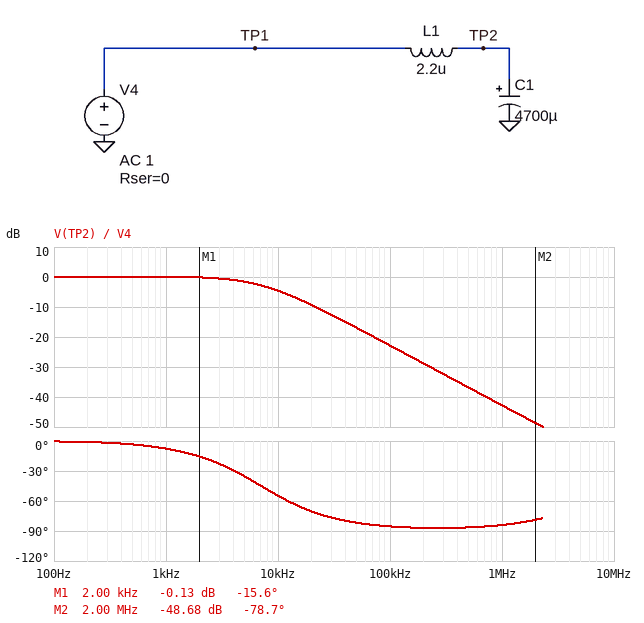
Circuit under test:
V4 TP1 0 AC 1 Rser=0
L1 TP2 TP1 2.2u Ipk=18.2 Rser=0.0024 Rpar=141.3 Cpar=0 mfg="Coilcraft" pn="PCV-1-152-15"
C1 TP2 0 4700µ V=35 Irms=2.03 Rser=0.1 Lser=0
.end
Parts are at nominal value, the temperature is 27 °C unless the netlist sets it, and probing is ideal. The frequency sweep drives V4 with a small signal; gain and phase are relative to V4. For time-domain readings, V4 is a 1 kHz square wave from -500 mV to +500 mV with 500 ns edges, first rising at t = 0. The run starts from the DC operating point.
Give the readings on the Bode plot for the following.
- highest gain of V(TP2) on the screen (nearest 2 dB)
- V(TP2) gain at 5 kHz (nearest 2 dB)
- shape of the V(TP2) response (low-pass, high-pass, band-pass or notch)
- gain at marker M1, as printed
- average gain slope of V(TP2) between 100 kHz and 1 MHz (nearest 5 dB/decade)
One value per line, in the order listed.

0 dB
-2 dB
low-pass
-0.13 dB
-20 dB/decade
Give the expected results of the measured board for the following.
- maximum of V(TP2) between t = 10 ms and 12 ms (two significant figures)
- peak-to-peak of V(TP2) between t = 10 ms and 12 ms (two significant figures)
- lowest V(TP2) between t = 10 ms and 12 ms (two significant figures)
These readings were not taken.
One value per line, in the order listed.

510 mV
1.0 V
-510 mV
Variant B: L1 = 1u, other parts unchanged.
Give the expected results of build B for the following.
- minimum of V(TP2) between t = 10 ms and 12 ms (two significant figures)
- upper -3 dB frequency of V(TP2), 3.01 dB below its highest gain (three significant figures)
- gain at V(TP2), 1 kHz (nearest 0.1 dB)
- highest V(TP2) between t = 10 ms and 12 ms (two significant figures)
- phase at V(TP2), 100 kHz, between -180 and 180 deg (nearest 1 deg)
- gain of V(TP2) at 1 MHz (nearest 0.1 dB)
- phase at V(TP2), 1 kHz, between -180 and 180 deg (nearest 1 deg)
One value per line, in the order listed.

-500 mV
15.9 kHz
0 dB
500 mV
-81 deg
-36.0 dB
-4 deg
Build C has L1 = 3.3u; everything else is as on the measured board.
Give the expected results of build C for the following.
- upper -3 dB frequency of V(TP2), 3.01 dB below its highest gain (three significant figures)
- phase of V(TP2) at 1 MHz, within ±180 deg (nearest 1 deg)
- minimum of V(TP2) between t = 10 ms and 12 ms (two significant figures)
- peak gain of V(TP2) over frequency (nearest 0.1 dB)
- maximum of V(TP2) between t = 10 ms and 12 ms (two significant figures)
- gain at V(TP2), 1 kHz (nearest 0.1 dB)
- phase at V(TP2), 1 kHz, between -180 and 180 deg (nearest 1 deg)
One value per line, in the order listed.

4.77 kHz
-81 deg
-520 mV
0.3 dB
520 mV
0.2 dB
-11 deg
